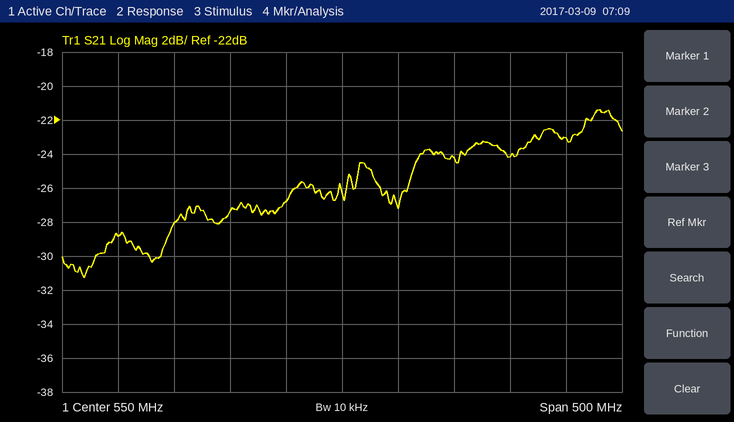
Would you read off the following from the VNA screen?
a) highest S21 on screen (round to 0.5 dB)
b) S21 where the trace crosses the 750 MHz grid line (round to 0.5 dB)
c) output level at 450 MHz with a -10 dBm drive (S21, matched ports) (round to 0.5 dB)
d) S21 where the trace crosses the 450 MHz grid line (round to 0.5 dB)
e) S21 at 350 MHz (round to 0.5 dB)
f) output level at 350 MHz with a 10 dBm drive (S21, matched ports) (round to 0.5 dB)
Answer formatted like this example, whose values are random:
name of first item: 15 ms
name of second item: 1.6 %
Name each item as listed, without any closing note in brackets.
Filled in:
highest S21 on screen: -21.5 dB
S21 where the trace crosses the 750 MHz grid line: -23.0 dB
output level at 450 MHz with a -10 dBm drive (S21, matched ports): -37.5 dBm
S21 where the trace crosses the 450 MHz grid line: -27.5 dB
S21 at 350 MHz: -29.0 dB
output level at 350 MHz with a 10 dBm drive (S21, matched ports): -19.0 dBm
